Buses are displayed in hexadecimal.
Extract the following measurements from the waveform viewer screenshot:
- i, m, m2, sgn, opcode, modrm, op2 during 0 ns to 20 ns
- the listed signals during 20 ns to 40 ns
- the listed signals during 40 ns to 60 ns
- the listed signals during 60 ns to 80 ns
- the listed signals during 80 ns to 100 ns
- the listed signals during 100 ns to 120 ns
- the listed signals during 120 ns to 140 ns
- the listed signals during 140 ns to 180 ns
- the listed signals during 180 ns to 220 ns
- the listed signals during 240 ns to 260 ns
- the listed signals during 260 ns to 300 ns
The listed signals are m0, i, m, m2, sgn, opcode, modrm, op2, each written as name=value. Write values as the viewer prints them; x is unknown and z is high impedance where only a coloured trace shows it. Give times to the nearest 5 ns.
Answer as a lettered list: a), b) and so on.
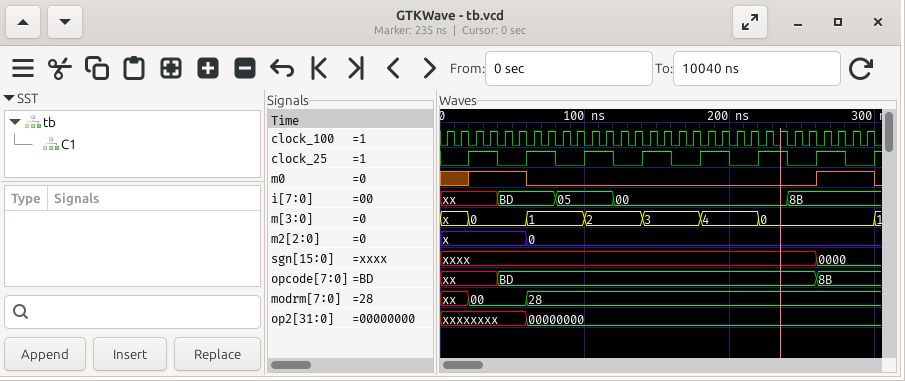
a) i=xx, m=x, m2=x, sgn=xxxx, opcode=xx, modrm=xx, op2=xxxxxxxx
b) m0=1, i=xx, m=0, m2=x, sgn=xxxx, opcode=xx, modrm=00, op2=xxxxxxxx
c) m0=1, i=BD, m=0, m2=x, sgn=xxxx, opcode=BD, modrm=00, op2=xxxxxxxx
d) m0=0, i=BD, m=1, m2=0, sgn=xxxx, opcode=BD, modrm=28, op2=00000000
e) m0=0, i=05, m=1, m2=0, sgn=xxxx, opcode=BD, modrm=28, op2=00000000
f) m0=0, i=05, m=2, m2=0, sgn=xxxx, opcode=BD, modrm=28, op2=00000000
g) m0=0, i=00, m=2, m2=0, sgn=xxxx, opcode=BD, modrm=28, op2=00000000
h) m0=0, i=00, m=3, m2=0, sgn=xxxx, opcode=BD, modrm=28, op2=00000000
i) m0=0, i=00, m=4, m2=0, sgn=xxxx, opcode=BD, modrm=28, op2=00000000
j) m0=0, i=8B, m=0, m2=0, sgn=xxxx, opcode=BD, modrm=28, op2=00000000
k) m0=1, i=8B, m=0, m2=0, sgn=0000, opcode=8B, modrm=28, op2=00000000
